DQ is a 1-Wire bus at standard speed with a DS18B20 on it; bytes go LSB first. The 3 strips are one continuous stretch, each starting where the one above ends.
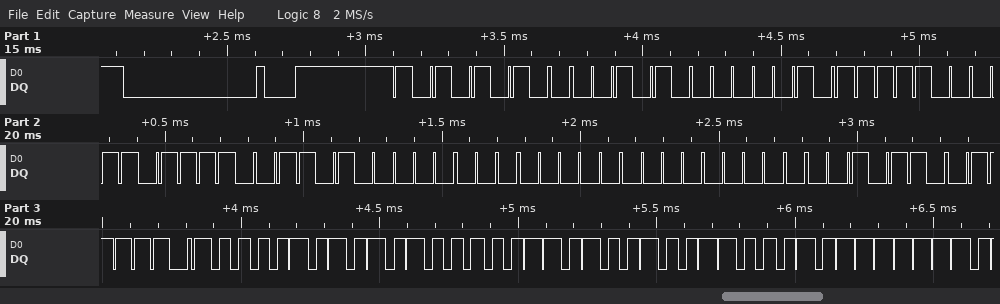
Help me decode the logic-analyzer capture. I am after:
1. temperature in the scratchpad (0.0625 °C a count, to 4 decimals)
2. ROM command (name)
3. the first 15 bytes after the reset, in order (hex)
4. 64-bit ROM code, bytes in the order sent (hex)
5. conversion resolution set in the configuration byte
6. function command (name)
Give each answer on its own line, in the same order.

85.0000 °C
Match ROM
55 28 D0 C7 9E 05 00 00 68 BE 50 05 4B 46 7F
28 D0 C7 9E 05 00 00 68
12 bits
Read Scratchpad
